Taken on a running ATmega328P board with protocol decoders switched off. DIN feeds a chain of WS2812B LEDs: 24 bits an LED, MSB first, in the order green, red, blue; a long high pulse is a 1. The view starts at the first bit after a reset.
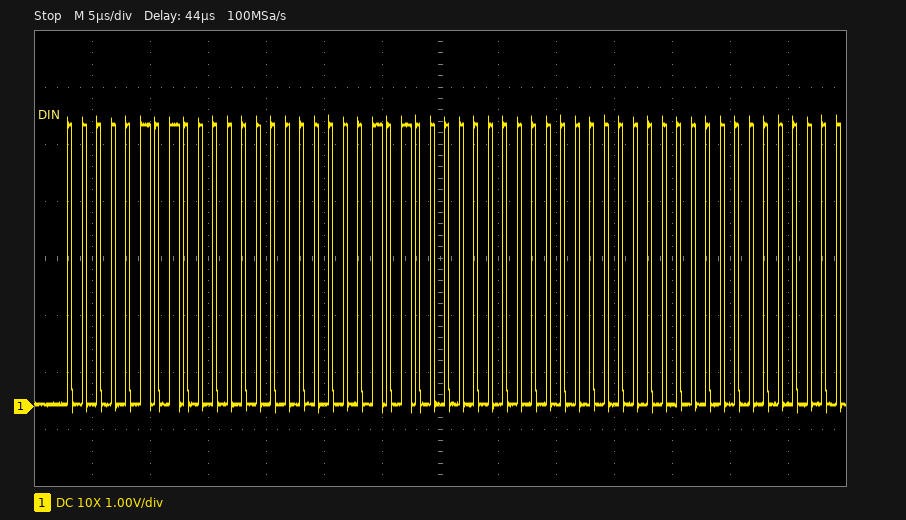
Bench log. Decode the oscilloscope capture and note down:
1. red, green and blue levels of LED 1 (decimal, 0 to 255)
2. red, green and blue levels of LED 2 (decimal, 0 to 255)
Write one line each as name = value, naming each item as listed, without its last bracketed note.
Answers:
red, green and blue levels of LED 1 = 0, 5, 5
red, green and blue levels of LED 2 = 0, 0, 0
